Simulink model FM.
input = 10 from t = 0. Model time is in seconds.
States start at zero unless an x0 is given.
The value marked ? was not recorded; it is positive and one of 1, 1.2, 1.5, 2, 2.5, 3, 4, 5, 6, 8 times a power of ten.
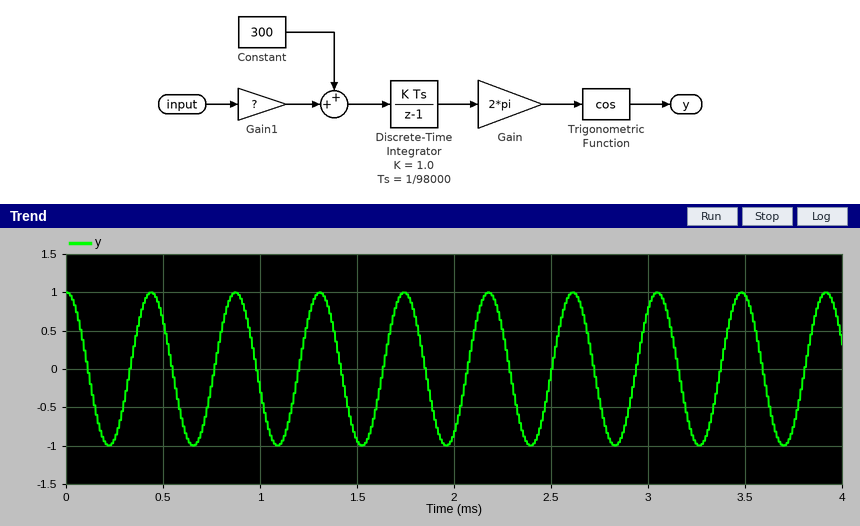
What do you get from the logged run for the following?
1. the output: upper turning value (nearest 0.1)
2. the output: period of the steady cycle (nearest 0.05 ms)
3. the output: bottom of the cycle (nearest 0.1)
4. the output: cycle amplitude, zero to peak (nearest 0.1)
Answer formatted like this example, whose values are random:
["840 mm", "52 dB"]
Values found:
["1.0", "0.45 ms", "-1.0", "1.0"]
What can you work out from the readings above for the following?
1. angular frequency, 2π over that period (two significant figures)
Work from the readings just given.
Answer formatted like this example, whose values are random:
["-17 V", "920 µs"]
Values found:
["14 rad/ms"]
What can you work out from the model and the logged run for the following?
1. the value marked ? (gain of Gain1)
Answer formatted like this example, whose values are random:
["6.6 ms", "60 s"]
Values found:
["200"]
